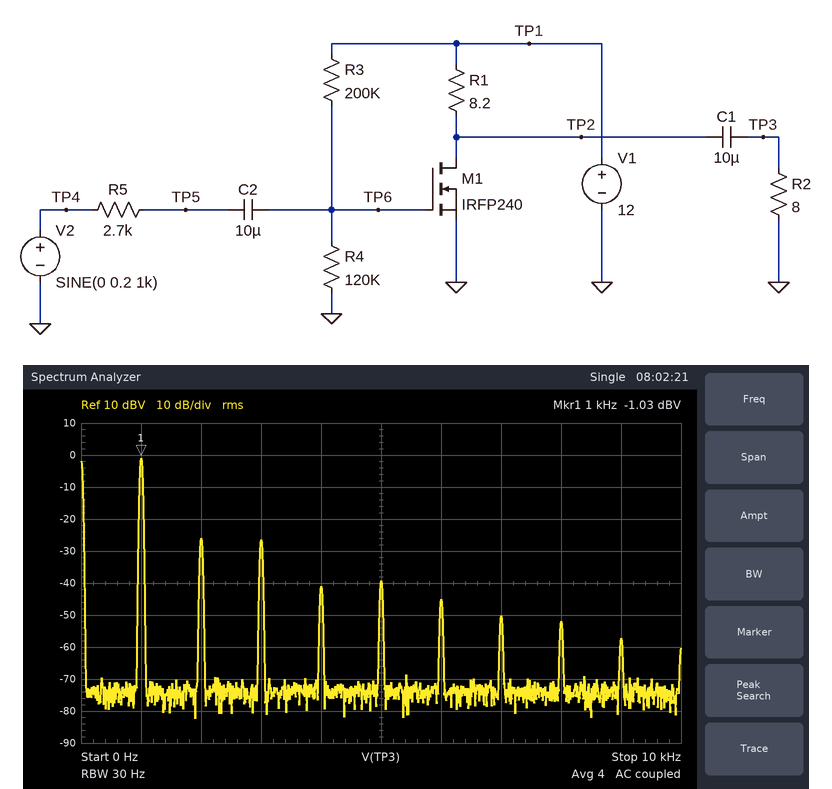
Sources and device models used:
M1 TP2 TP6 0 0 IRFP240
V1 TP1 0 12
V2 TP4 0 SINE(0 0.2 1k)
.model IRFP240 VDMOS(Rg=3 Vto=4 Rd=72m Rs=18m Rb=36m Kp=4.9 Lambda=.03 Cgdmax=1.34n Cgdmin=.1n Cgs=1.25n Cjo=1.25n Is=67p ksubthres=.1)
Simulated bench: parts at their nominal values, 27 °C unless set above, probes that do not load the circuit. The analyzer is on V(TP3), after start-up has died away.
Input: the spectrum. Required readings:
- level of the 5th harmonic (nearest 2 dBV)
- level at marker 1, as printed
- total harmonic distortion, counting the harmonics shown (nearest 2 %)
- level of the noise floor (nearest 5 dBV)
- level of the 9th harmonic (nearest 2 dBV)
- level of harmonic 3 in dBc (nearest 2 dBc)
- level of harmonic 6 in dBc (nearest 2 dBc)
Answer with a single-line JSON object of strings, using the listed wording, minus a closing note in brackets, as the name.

{"level of the 5th harmonic": "-40 dBV", "level at marker 1, as printed": "-1.03 dBV", "total harmonic distortion, counting the harmonics shown": "8 %", "level of the noise floor": "-75 dBV", "level of the 9th harmonic": "-58 dBV", "level of harmonic 3 in dBc": "-26 dBc", "level of harmonic 6 in dBc": "-44 dBc"}
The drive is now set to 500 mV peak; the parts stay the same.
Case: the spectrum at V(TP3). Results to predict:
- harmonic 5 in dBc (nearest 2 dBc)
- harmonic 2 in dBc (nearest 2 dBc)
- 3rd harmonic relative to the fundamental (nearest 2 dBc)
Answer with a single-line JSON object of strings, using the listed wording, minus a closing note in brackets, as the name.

{"harmonic 5 in dBc": "-34 dBc", "harmonic 2 in dBc": "-44 dBc", "3rd harmonic relative to the fundamental": "-16 dBc"}
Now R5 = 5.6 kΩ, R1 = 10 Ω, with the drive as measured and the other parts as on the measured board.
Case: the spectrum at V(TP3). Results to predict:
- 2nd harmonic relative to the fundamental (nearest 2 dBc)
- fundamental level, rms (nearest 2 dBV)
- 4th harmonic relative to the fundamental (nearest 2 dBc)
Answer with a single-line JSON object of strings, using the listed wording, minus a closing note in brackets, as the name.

{"2nd harmonic relative to the fundamental": "-16 dBc", "fundamental level, rms": "-2 dBV", "4th harmonic relative to the fundamental": "-28 dBc"}
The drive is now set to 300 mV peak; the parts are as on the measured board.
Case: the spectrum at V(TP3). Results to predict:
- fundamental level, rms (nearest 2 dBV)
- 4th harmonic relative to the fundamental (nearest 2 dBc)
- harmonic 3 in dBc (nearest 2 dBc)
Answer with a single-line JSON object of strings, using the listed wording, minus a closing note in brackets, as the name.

{"fundamental level, rms": "2 dBV", "4th harmonic relative to the fundamental": "-32 dBc", "harmonic 3 in dBc": "-24 dBc"}
